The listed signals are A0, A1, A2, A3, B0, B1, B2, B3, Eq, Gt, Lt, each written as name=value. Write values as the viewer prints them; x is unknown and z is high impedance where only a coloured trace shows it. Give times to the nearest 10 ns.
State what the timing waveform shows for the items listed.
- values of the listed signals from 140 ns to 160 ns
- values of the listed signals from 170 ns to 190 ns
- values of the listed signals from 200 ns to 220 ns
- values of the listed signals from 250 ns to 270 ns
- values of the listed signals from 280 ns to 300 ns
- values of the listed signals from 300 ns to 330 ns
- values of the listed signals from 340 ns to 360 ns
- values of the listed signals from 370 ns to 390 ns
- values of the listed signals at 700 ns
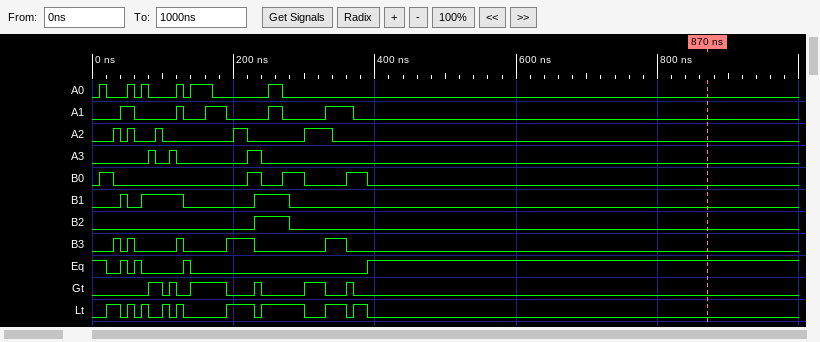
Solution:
A0=1, A1=0, A2=0, A3=0, B0=0, B1=0, B2=0, B3=0, Eq=0, Gt=1, Lt=0
A0=0, A1=1, A2=0, A3=0, B0=0, B1=0, B2=0, B3=0, Eq=0, Gt=1, Lt=0
A0=0, A1=0, A2=1, A3=0, B0=0, B1=0, B2=0, B3=1, Eq=0, Gt=0, Lt=1
A0=1, A1=1, A2=0, A3=0, B0=0, B1=1, B2=1, B3=0, Eq=0, Gt=0, Lt=1
A0=0, A1=0, A2=0, A3=0, B0=1, B1=0, B2=0, B3=0, Eq=0, Gt=0, Lt=1
A0=0, A1=0, A2=1, A3=0, B0=0, B1=0, B2=0, B3=0, Eq=0, Gt=1, Lt=0
A0=0, A1=1, A2=0, A3=0, B0=0, B1=0, B2=0, B3=1, Eq=0, Gt=0, Lt=1
A0=0, A1=0, A2=0, A3=0, B0=1, B1=0, B2=0, B3=0, Eq=0, Gt=0, Lt=1
A0=0, A1=0, A2=0, A3=0, B0=0, B1=0, B2=0, B3=0, Eq=1, Gt=0, Lt=0
